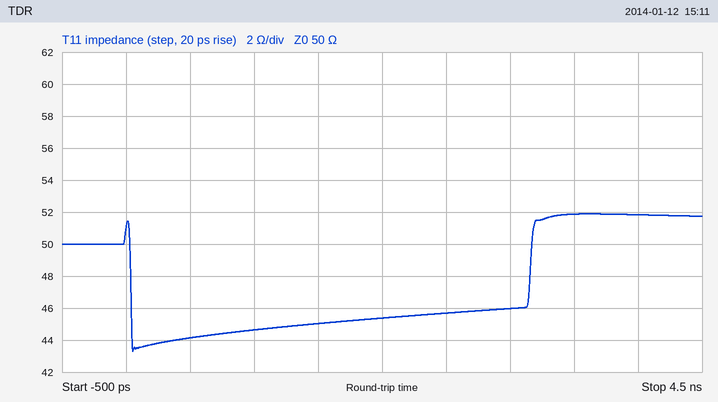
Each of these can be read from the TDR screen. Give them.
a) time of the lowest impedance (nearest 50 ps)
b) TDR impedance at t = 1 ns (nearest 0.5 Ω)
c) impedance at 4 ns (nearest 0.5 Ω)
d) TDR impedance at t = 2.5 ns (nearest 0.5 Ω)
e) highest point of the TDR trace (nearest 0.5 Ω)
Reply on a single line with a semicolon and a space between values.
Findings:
50 ps; 44.5 Ω; 52.0 Ω; 45.5 Ω; 52.0 Ω
